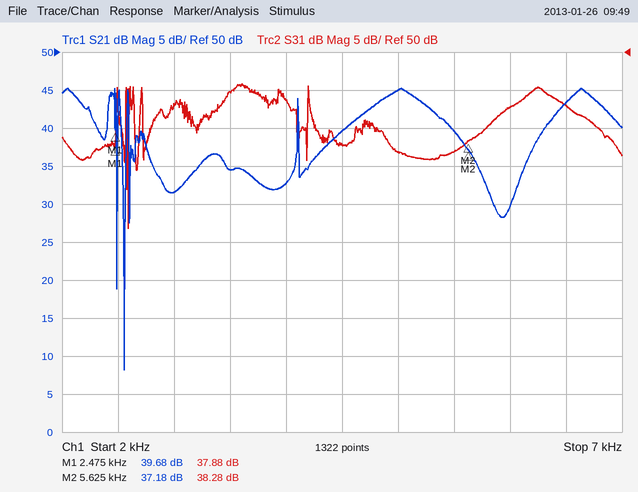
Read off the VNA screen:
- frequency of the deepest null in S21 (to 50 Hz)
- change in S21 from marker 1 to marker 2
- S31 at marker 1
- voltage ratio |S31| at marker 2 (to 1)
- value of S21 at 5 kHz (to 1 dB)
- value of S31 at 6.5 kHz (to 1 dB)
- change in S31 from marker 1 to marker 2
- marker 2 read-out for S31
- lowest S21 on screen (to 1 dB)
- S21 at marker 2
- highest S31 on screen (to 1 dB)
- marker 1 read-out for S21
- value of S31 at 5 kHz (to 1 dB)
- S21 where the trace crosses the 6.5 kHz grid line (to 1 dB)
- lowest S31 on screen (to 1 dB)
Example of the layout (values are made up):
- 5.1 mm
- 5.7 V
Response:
- 2.55 kHz
- -2.50 dB
- 37.88 dB
- 82
- 45 dB
- 43 dB
- 0.40 dB
- 38.28 dB
- 8 dB
- 37.18 dB
- 46 dB
- 39.68 dB
- 37 dB
- 43 dB
- 27 dB
